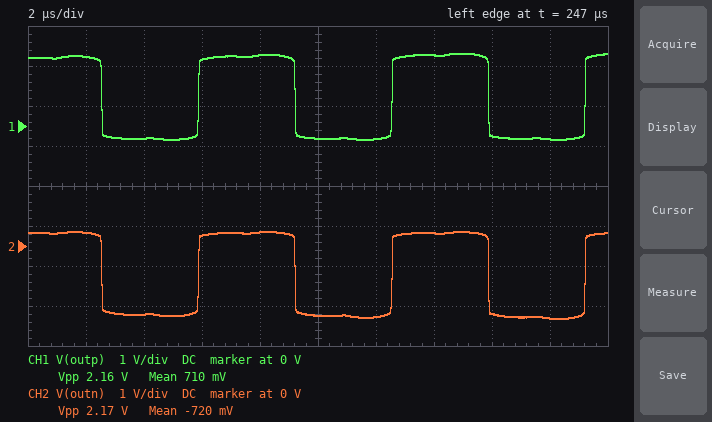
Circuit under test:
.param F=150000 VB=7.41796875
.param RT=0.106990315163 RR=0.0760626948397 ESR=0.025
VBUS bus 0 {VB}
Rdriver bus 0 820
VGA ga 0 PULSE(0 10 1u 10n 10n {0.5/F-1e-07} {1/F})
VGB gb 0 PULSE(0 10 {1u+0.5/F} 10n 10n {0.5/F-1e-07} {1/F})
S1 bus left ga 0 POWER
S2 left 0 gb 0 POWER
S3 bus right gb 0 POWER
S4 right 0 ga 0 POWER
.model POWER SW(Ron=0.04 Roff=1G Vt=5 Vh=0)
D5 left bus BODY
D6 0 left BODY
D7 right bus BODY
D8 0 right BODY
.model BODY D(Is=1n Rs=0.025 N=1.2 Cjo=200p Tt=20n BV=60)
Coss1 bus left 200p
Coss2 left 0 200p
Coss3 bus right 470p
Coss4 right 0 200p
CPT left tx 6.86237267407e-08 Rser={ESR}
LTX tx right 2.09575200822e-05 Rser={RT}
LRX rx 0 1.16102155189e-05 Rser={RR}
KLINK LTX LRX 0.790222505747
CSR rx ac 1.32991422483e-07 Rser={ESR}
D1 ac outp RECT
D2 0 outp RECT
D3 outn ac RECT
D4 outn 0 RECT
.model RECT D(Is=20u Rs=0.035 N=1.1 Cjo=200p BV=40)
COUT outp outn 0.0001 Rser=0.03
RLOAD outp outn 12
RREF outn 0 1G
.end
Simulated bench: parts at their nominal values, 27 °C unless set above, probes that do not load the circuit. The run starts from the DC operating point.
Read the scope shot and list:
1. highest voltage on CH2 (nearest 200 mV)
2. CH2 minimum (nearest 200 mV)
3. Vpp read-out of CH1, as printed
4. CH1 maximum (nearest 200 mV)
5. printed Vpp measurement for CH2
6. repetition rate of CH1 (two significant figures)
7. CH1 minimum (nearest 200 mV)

400 mV
-1.8 V
2.16 V
1.8 V
2.17 V
150 kHz
-400 mV
